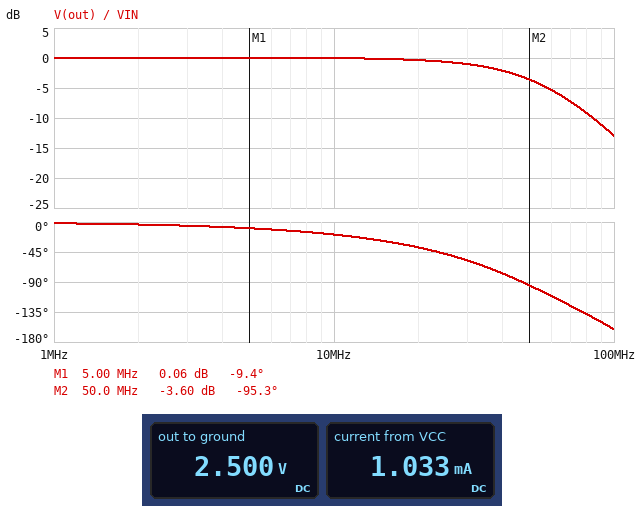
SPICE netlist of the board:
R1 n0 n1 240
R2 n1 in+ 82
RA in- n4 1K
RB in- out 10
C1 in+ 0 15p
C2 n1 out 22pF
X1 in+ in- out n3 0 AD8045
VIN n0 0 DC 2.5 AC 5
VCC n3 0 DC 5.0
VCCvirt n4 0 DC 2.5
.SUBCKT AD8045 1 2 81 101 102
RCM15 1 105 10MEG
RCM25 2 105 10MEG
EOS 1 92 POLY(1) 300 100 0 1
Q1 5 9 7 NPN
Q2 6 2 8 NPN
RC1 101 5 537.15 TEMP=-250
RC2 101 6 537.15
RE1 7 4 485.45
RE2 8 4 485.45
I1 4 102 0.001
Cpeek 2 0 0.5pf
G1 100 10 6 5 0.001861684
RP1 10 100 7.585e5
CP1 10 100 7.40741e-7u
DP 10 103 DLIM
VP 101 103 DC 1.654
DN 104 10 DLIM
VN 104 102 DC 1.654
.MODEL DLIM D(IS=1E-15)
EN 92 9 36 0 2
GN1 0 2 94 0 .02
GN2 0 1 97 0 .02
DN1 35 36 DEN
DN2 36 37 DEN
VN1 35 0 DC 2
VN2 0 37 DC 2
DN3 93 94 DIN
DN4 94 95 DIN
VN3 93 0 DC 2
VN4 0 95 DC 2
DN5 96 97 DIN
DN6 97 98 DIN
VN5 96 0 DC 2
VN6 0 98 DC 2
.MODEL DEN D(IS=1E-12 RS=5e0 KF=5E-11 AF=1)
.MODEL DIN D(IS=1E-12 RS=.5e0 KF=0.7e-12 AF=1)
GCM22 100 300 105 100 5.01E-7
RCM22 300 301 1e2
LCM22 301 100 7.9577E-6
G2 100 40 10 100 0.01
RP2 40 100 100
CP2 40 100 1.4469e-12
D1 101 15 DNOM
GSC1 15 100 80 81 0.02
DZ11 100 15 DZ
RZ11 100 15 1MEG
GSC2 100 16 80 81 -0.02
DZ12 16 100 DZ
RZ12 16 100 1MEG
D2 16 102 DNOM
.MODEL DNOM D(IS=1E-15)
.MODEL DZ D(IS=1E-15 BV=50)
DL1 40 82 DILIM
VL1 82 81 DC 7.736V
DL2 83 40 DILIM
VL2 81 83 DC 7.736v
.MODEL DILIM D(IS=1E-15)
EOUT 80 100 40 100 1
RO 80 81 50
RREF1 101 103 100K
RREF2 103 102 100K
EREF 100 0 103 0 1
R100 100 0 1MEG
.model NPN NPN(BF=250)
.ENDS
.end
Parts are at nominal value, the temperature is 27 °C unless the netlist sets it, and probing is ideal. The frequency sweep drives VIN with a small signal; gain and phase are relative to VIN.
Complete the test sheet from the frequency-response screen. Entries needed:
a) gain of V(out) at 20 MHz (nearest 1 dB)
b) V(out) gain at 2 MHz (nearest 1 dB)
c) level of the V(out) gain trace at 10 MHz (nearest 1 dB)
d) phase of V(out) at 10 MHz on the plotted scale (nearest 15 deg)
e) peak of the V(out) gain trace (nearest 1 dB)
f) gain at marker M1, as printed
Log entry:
0 dB
0 dB
0 dB
-15 deg
0 dB
0.06 dB
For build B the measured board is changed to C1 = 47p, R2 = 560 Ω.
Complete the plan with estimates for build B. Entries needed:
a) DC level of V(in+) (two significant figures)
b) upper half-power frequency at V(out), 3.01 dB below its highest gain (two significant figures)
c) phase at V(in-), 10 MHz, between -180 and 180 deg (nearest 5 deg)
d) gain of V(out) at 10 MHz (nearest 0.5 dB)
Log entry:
2.5 V
4.7 MHz
-80 deg
-7.5 dB
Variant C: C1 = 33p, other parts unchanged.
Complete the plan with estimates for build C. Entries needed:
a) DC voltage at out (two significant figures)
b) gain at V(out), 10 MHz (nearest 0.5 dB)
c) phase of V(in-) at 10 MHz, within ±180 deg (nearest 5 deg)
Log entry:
2.5 V
-1.0 dB
-35 deg
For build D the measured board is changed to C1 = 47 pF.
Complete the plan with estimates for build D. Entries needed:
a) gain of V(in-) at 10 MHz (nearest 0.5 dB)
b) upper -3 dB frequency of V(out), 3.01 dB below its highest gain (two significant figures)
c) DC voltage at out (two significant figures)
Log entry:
-2.5 dB
12 MHz
2.5 V
